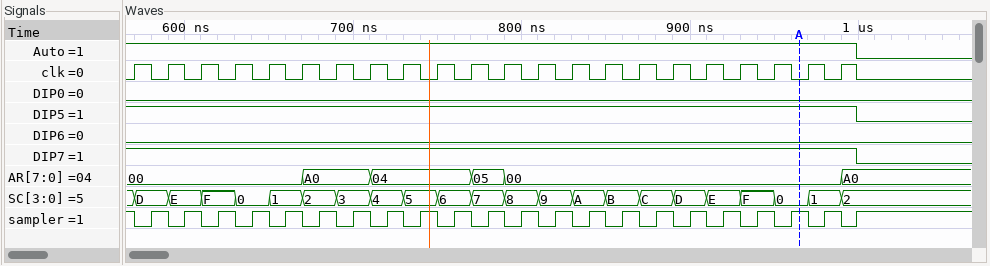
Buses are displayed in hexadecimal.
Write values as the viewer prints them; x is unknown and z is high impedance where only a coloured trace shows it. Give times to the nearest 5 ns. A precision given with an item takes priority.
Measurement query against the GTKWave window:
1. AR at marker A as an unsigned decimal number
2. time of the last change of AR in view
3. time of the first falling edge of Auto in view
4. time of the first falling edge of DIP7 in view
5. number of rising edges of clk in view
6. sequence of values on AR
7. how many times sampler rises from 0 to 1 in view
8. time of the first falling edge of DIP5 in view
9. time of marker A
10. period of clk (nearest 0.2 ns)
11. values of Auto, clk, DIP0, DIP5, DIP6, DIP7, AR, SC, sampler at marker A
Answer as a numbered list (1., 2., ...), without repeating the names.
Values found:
1. 0
2. 990 ns
3. 1000 ns
4. 1000 ns
5. 22
6. 00, A0, 04, 05, 00, A0
7. 22
8. 1000 ns
9. 965 ns
10. 20 ns
11. Auto=1, clk=0, DIP0=0, DIP5=1, DIP6=0, DIP7=1, AR=00, SC=0, sampler=1
